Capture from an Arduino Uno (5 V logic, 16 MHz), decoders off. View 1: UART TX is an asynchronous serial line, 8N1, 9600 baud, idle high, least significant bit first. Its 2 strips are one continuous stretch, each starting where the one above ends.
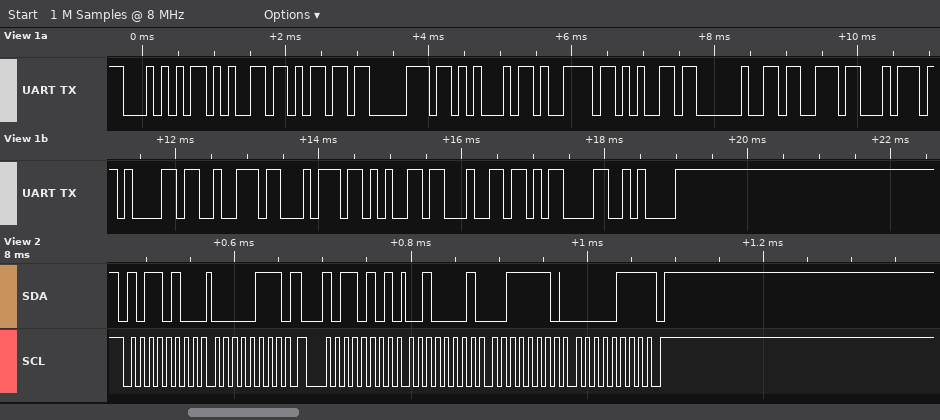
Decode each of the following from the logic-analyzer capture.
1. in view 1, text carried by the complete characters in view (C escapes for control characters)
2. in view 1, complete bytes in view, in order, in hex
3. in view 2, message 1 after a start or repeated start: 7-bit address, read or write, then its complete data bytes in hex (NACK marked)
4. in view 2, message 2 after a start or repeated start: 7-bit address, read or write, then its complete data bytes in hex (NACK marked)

"TempEye started\r\n"
54 65 6D 70 45 79 65 20 73 74 61 72 74 65 64 0D 0A
0x5A write: 07
0x5A read: 21 3E 07 NACK
